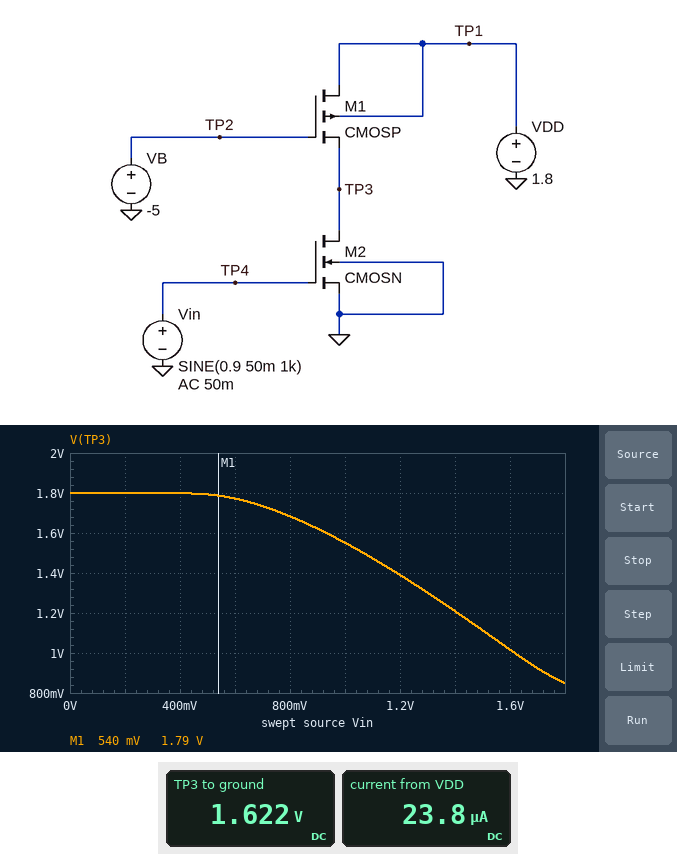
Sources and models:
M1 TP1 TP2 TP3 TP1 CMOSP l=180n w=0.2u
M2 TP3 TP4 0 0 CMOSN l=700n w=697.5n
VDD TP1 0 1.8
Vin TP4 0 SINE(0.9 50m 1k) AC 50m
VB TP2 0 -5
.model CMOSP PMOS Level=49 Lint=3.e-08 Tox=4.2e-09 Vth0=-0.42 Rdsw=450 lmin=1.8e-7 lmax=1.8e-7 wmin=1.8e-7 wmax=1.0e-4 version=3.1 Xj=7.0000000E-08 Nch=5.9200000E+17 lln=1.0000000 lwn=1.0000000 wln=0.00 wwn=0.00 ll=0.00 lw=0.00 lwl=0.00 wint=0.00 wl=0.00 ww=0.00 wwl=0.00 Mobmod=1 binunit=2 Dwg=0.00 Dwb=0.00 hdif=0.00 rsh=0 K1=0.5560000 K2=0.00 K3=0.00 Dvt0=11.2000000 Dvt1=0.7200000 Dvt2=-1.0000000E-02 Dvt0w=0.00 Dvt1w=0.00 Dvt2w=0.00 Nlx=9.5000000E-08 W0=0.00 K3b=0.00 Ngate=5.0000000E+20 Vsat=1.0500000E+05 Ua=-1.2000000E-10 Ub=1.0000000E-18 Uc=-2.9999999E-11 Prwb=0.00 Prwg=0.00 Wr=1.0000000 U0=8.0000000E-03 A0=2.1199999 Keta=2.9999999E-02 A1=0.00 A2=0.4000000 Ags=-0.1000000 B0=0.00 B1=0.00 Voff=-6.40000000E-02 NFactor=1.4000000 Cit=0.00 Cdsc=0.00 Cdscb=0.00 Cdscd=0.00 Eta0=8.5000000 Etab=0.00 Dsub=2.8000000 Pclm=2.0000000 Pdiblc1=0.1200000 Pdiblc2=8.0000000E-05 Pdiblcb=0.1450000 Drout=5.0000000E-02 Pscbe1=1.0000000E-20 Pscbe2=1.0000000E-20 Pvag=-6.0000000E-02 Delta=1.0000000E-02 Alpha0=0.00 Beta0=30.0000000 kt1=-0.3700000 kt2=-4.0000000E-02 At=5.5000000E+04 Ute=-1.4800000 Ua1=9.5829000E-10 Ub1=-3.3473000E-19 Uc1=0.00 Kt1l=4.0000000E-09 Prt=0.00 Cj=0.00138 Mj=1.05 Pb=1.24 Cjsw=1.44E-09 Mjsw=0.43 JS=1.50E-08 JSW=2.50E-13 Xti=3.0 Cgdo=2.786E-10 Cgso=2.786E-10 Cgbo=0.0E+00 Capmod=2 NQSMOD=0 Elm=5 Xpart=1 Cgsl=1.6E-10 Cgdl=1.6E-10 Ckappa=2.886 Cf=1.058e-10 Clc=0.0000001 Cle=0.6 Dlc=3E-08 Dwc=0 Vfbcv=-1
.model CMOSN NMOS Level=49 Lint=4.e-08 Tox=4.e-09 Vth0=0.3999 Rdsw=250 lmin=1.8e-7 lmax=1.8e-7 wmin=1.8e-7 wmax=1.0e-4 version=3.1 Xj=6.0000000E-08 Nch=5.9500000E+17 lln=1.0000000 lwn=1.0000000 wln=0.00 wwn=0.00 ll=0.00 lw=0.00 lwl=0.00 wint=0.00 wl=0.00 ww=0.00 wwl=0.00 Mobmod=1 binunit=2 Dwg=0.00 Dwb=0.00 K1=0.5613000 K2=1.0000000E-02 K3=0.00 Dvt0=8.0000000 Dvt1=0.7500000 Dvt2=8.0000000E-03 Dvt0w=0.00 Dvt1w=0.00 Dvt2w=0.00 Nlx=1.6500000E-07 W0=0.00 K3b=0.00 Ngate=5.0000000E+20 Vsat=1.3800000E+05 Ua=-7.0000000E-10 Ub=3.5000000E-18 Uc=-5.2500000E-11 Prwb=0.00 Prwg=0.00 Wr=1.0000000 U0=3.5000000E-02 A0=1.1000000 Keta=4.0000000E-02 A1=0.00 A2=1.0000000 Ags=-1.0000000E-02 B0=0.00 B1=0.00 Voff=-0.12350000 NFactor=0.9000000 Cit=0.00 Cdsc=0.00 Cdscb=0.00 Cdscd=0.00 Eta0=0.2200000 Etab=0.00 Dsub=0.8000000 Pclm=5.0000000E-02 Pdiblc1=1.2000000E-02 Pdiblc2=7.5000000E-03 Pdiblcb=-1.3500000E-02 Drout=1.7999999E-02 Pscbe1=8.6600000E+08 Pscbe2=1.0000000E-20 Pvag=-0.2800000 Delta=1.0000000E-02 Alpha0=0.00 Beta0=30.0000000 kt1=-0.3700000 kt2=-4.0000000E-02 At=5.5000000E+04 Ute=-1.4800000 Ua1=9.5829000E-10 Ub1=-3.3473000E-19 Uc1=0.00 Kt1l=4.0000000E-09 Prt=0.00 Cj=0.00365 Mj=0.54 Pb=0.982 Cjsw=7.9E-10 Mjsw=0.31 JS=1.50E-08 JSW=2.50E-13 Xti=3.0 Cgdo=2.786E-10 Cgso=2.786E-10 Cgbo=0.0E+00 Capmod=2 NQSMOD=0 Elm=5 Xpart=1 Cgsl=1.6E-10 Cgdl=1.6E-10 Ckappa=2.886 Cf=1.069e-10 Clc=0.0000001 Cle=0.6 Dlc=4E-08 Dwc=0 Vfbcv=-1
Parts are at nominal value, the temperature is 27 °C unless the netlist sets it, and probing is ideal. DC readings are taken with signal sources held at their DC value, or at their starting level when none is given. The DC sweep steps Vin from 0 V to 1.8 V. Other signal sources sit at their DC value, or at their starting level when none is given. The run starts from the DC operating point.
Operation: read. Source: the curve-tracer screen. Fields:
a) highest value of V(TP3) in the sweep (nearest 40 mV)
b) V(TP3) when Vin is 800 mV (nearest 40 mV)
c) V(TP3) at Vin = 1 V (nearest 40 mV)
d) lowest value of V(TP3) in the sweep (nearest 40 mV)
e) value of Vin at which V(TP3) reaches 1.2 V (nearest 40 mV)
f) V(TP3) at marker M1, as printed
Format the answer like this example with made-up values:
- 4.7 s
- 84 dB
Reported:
- 1.80 V
- 1.68 V
- 1.56 V
- 840 mV
- 1.40 V
- 1.79 V
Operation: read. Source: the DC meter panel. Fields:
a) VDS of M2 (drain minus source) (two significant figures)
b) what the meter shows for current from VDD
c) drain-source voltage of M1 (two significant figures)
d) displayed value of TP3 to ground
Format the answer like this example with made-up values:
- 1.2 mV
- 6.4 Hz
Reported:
- 1.6 V
- 23.8 µA
- 180 mV
- 1.622 V
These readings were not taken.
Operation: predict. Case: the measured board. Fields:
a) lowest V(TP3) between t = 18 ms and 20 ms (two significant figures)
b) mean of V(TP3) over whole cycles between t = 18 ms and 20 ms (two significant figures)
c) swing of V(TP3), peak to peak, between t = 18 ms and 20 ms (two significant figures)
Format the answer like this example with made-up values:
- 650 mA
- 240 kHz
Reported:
- 1.6 V
- 1.6 V
- 66 mV
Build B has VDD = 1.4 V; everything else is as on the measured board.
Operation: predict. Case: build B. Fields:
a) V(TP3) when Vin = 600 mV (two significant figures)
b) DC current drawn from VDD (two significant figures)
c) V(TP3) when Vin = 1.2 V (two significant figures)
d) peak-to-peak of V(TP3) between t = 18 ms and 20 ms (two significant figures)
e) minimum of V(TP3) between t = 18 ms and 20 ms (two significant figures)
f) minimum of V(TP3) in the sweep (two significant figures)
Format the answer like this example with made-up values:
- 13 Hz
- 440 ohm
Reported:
- 1.4 V
- 23 µA
- 1.0 V
- 64 mV
- 1.2 V
- 600 mV
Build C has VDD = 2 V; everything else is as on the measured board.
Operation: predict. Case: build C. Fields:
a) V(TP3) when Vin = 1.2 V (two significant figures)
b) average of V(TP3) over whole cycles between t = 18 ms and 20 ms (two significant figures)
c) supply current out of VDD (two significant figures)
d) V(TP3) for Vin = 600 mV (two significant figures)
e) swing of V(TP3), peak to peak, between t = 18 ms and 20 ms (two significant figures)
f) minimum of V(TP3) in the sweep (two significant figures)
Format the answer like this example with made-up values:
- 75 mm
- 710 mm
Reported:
- 1.6 V
- 1.8 V
- 24 µA
- 2.0 V
- 67 mV
- 1.0 V
